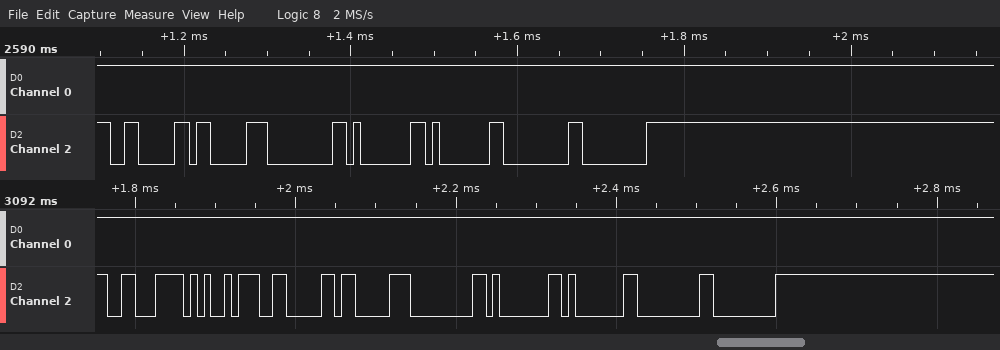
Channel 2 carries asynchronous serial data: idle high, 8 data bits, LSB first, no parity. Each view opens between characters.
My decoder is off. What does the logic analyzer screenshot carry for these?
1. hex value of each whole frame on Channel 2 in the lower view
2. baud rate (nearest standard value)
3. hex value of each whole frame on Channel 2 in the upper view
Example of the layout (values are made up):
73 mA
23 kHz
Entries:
C6, A5, 06, 83, 00, 01, 01, 00, 00
115200 baud
06, 83, 00, 01, 01, 00, 00
